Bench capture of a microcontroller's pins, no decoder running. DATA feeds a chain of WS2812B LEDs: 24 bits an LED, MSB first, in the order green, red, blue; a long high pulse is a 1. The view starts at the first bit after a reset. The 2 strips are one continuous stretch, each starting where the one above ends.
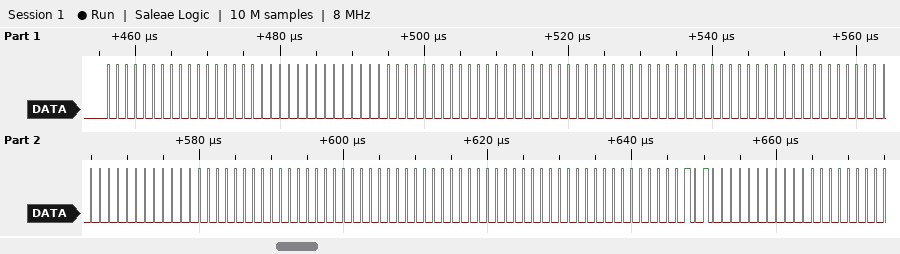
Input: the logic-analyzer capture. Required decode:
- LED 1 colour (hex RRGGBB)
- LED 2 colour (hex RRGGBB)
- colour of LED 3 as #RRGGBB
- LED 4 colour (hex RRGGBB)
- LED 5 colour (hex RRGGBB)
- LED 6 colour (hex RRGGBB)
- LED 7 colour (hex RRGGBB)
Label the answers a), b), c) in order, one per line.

a) #000000
b) #000000
c) #000000
d) #000000
e) #000000
f) #000000
g) #500000
